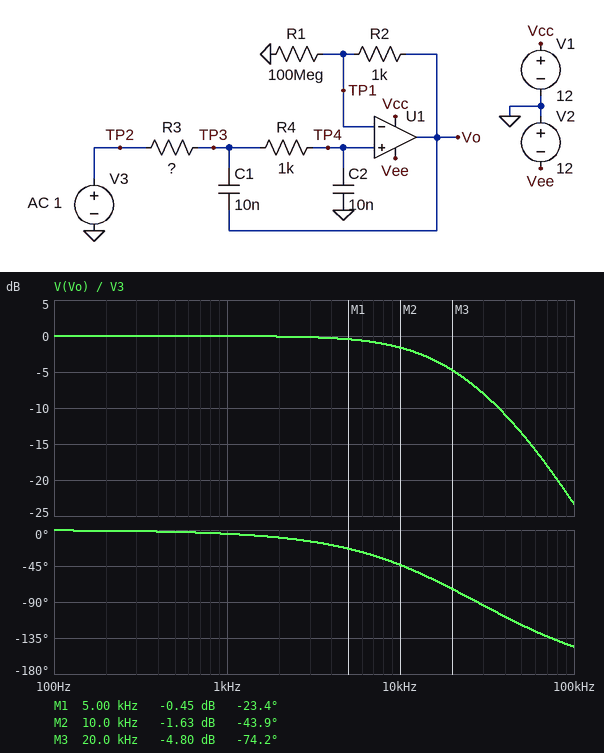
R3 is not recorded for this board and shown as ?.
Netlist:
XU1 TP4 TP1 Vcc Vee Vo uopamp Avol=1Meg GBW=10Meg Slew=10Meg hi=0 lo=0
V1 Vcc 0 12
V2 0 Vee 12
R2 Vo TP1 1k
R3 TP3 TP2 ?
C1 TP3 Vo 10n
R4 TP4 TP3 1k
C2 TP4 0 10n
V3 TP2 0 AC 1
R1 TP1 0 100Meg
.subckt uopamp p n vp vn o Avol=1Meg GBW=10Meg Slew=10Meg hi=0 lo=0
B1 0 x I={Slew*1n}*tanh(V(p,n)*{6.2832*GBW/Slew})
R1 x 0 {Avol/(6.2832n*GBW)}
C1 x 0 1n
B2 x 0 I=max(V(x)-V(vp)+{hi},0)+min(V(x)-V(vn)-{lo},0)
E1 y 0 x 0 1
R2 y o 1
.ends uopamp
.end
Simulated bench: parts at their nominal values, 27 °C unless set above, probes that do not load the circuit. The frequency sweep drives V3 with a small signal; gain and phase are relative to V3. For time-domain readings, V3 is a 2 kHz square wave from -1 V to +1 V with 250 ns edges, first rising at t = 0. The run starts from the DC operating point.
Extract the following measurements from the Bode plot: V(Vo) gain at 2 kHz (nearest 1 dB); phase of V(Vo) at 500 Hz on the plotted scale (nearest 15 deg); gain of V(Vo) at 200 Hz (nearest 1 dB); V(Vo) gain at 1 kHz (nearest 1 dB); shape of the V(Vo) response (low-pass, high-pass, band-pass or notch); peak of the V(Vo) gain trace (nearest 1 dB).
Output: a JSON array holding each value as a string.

["0 dB", "0 deg", "0 dB", "0 dB", "low-pass", "0 dB"]
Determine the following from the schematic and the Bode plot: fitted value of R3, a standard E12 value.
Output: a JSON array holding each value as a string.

["330 Ω"]
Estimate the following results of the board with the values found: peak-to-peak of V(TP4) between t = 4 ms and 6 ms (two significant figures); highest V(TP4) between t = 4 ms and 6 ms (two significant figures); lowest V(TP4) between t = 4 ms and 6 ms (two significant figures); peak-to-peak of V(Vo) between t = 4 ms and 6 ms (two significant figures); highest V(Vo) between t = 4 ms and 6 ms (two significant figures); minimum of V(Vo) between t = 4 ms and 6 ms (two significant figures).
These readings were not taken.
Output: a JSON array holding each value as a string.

["2.0 V", "1.0 V", "-1.0 V", "2.0 V", "1.0 V", "-1.0 V"]
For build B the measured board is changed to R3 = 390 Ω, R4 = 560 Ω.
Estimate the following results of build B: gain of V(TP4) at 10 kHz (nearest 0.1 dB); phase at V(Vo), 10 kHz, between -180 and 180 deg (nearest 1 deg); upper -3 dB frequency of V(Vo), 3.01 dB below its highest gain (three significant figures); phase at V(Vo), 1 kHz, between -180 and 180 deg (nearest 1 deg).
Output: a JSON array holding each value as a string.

["-0.8 dB", "-33 deg", "21.4 kHz", "-3 deg"]
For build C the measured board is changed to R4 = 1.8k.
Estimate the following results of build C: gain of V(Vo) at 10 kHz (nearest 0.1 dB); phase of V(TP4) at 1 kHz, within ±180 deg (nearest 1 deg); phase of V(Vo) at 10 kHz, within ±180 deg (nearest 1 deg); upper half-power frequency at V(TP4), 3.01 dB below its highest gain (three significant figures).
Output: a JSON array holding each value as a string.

["-3.8 dB", "-8 deg", "-60 deg", "8.57 kHz"]
